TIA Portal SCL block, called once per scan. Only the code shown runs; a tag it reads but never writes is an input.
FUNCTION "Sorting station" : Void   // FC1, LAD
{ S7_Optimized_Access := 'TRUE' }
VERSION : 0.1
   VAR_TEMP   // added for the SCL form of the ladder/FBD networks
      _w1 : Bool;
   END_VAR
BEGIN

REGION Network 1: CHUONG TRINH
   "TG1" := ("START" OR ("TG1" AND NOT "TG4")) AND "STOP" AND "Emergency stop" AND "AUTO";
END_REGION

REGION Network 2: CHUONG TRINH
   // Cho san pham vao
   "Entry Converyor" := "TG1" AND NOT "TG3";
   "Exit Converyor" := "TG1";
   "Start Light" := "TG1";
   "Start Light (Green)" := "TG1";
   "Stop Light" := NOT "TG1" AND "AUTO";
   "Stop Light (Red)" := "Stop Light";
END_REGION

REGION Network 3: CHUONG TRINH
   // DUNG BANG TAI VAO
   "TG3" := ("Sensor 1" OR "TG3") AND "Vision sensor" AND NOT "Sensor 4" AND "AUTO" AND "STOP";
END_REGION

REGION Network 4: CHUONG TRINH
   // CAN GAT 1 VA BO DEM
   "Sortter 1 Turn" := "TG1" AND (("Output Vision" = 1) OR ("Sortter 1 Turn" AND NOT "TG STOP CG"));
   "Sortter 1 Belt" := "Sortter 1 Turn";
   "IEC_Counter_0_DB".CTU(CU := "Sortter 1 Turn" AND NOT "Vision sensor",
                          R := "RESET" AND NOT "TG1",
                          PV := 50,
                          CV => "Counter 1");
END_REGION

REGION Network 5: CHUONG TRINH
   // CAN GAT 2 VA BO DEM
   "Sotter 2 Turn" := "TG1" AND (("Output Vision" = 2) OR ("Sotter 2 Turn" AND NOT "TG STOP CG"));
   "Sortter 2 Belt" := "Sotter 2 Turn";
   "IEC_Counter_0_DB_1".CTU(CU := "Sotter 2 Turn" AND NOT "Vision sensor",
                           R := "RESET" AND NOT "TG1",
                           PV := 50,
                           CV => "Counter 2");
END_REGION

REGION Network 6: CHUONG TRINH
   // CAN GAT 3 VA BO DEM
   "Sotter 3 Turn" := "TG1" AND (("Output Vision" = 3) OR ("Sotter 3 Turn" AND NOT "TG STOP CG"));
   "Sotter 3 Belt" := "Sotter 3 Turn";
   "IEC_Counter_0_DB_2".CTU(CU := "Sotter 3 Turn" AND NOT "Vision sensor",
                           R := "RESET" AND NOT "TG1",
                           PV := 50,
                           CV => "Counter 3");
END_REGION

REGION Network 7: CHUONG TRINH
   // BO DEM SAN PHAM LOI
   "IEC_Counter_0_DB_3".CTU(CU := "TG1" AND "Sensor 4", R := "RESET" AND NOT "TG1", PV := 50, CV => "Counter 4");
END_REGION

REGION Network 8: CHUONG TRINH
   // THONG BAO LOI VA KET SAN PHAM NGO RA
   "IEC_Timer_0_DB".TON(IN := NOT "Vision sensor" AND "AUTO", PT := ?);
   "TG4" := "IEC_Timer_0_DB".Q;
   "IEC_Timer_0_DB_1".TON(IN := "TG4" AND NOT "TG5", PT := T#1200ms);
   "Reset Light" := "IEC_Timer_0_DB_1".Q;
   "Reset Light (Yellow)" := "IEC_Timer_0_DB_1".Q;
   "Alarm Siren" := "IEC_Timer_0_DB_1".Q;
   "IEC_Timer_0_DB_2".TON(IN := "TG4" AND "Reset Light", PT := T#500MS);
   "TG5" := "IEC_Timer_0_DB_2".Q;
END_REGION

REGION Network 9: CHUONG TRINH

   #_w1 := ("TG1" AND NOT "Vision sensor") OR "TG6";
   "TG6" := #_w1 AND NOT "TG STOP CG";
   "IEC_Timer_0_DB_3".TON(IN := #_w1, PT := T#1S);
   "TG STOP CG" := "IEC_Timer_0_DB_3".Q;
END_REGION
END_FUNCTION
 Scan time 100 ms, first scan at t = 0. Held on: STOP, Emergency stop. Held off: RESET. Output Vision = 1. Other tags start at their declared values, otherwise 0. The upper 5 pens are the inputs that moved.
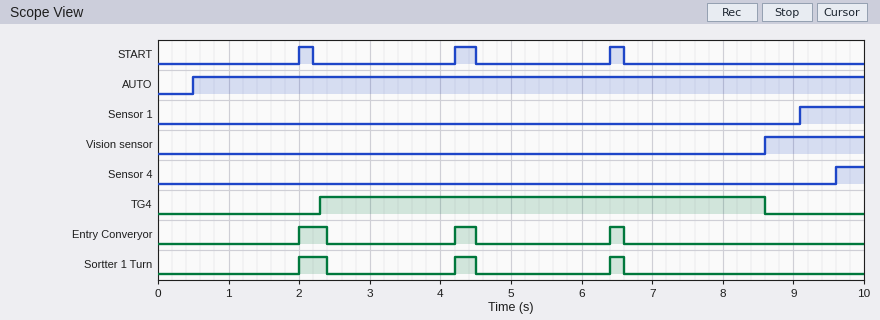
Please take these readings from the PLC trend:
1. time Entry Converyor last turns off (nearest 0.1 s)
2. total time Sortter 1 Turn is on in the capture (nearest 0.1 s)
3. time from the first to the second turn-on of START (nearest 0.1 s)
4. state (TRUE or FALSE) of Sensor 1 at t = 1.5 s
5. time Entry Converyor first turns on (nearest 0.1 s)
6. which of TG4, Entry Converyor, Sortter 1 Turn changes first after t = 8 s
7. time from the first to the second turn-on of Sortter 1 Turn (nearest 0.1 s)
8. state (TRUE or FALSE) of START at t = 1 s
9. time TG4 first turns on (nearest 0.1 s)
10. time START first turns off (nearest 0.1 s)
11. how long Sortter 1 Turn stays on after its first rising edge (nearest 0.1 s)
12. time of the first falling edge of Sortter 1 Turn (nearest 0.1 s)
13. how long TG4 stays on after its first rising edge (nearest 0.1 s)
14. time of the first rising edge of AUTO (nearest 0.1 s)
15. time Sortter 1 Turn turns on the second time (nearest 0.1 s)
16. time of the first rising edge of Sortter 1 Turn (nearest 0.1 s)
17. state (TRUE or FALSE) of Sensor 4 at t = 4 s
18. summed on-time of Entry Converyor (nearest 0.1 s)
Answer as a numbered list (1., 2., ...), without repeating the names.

1. 6.6 s
2. 0.9 s
3. 2.2 s
4. FALSE
5. 2.0 s
6. TG4
7. 2.2 s
8. FALSE
9. 2.3 s
10. 2.2 s
11. 0.4 s
12. 2.4 s
13. 6.3 s
14. 0.5 s
15. 4.2 s
16. 2.0 s
17. FALSE
18. 0.9 s
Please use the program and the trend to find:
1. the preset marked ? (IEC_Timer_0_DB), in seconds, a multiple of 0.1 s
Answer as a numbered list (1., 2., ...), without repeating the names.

1. 1.8 s
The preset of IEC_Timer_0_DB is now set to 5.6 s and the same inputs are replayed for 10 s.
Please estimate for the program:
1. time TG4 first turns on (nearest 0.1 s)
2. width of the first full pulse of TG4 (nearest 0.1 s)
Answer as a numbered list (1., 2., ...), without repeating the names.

1. 6.1 s
2. 2.5 s
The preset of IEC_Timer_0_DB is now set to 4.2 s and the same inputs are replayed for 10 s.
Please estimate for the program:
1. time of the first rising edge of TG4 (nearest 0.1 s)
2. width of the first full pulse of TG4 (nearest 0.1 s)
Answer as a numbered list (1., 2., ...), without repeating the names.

1. 4.7 s
2. 3.9 s
